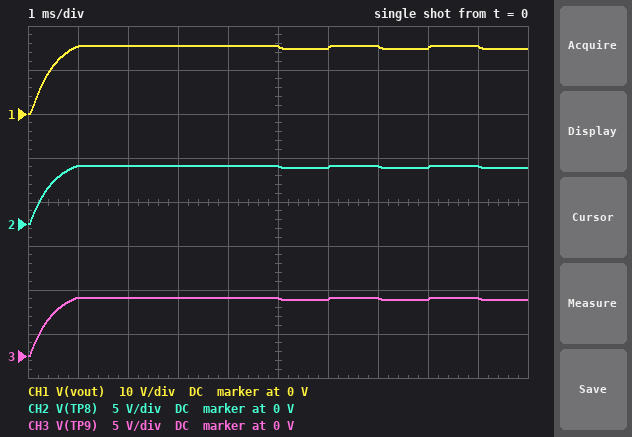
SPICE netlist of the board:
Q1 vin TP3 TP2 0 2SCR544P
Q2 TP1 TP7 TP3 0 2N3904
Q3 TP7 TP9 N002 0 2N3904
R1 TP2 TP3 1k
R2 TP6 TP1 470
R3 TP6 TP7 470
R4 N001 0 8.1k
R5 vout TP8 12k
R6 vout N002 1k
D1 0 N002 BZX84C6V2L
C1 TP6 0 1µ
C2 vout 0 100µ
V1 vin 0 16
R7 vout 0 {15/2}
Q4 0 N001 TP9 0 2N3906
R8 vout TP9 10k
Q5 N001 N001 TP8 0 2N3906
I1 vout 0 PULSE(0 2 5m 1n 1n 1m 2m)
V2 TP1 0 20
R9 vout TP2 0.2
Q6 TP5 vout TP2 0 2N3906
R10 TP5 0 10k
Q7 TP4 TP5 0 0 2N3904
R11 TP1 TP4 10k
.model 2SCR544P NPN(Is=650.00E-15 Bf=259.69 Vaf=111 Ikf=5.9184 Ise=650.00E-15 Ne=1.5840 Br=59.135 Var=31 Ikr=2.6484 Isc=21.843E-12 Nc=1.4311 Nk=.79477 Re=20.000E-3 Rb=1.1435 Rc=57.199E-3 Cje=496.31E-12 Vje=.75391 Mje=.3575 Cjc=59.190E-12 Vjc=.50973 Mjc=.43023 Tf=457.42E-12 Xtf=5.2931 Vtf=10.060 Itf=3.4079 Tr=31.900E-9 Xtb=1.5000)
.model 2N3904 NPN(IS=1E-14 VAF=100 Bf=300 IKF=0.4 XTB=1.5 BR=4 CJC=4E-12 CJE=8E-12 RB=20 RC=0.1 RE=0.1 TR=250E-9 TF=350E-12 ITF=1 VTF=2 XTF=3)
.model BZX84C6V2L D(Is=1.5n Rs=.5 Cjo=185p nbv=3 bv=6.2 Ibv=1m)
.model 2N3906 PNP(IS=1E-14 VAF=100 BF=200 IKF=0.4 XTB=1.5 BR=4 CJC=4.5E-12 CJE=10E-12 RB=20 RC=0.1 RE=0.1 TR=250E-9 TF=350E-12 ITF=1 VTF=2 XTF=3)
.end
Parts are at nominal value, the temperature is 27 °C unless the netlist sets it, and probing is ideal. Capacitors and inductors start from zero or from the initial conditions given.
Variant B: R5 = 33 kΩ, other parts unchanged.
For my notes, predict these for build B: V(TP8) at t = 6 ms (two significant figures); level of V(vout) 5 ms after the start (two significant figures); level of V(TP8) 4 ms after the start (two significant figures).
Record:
3.5 V
15 V
3.6 V
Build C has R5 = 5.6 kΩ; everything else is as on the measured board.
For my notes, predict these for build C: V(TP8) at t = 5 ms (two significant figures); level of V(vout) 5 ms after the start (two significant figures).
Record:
7.1 V
12 V
